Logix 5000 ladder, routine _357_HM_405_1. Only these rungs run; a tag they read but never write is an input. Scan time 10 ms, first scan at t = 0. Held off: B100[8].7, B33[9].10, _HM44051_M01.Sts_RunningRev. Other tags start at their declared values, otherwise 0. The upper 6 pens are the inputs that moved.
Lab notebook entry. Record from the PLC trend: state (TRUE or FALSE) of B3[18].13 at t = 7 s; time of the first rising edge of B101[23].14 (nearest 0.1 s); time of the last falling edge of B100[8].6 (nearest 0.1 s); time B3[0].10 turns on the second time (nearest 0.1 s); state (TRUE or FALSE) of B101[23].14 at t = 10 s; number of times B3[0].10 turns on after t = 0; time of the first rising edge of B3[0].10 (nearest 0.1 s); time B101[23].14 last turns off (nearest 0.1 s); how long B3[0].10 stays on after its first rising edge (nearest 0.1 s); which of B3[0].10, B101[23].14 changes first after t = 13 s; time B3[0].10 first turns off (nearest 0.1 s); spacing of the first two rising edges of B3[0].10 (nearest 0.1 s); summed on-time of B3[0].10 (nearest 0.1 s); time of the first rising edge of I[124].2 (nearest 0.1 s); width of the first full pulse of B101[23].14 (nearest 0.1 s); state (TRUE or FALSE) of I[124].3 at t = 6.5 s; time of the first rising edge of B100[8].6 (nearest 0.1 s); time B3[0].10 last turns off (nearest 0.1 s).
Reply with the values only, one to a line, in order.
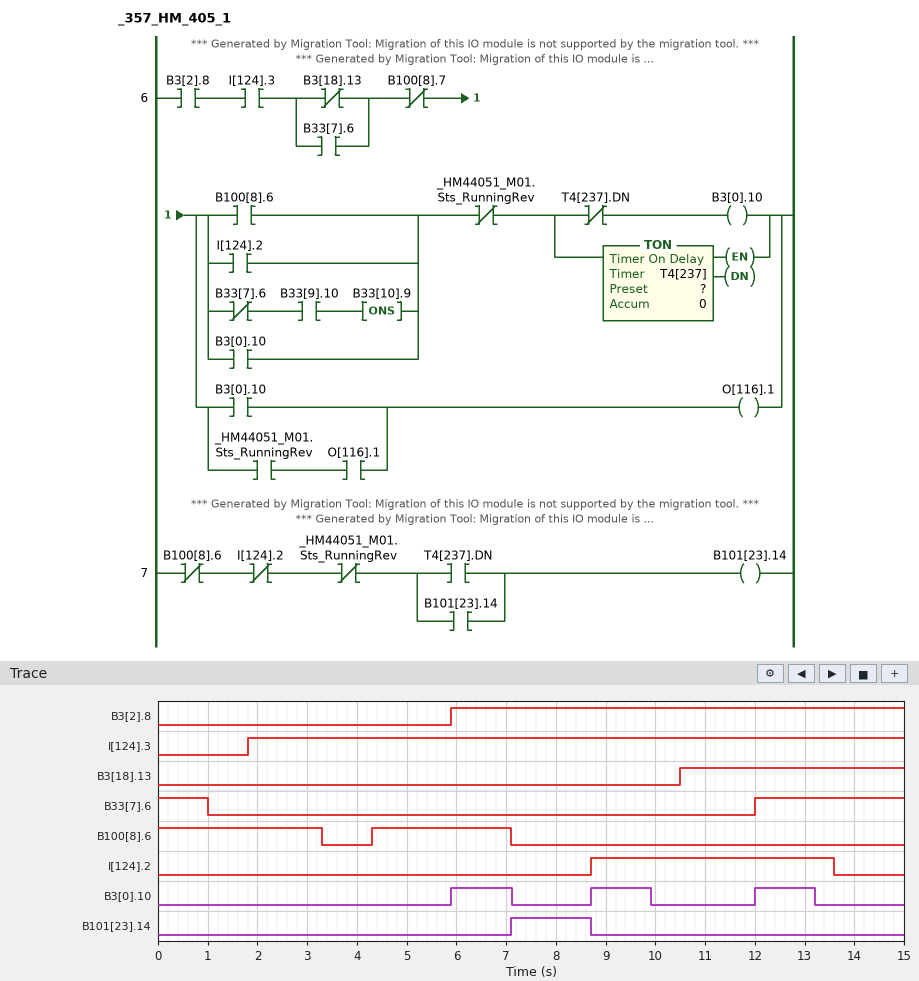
FALSE
7.1 s
7.1 s
8.7 s
FALSE
3
5.9 s
8.7 s
1.2 s
B3[0].10
7.1 s
2.8 s
3.6 s
8.7 s
1.6 s
TRUE
4.3 s
13.2 s
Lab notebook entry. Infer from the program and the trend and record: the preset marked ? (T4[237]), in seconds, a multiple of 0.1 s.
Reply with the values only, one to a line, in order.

1.2 s
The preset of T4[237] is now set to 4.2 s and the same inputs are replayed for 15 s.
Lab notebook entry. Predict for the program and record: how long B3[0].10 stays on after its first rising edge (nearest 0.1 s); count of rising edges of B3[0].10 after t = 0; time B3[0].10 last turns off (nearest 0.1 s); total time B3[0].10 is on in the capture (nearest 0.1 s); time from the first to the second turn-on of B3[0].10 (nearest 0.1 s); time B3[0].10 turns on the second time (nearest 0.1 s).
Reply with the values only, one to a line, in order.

4.2 s
2
10.1 s
7.2 s
6.1 s
12.0 s
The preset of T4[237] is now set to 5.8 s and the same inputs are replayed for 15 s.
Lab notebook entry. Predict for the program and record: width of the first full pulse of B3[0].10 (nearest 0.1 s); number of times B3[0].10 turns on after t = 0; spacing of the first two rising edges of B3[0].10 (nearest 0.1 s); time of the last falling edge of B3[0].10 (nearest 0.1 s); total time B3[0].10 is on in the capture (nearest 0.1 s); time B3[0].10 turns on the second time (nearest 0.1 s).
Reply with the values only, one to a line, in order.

4.6 s
2
6.1 s
10.5 s
7.6 s
12.0 s
